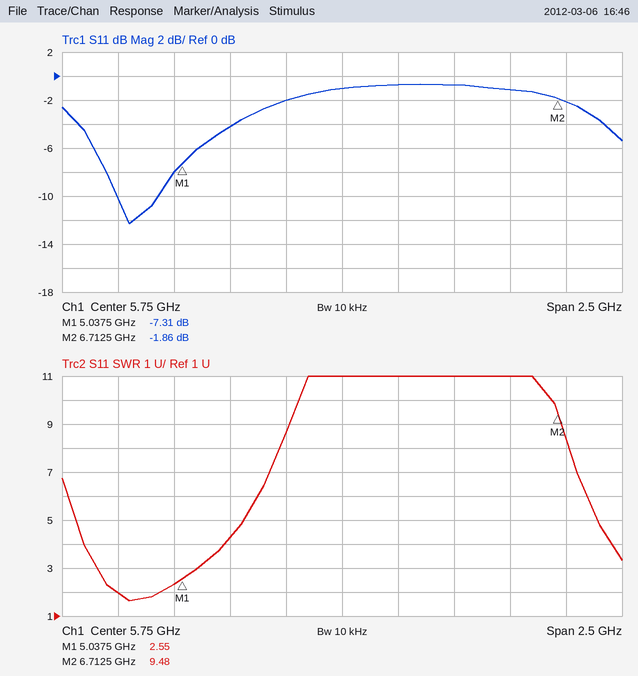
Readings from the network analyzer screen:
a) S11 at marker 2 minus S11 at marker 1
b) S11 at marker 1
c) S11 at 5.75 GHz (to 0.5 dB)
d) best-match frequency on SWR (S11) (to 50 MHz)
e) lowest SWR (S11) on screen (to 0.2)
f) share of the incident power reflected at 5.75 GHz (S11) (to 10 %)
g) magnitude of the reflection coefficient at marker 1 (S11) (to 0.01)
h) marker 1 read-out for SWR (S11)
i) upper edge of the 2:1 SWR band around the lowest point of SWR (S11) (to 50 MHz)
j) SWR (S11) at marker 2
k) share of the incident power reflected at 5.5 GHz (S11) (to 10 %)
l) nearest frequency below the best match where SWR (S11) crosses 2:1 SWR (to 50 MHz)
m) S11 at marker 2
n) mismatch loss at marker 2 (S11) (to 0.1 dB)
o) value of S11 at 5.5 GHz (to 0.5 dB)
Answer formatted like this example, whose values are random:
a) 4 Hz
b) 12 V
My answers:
a) 5.45 dB
b) -7.31 dB
c) -1.0 dB
d) 4.80 GHz
e) 1.6
f) 80 %
g) 0.43
h) 2.55
i) 4.95 GHz
j) 9.48
k) 60 %
l) 4.75 GHz
m) -1.86 dB
n) 4.6 dB
o) -2.0 dB
